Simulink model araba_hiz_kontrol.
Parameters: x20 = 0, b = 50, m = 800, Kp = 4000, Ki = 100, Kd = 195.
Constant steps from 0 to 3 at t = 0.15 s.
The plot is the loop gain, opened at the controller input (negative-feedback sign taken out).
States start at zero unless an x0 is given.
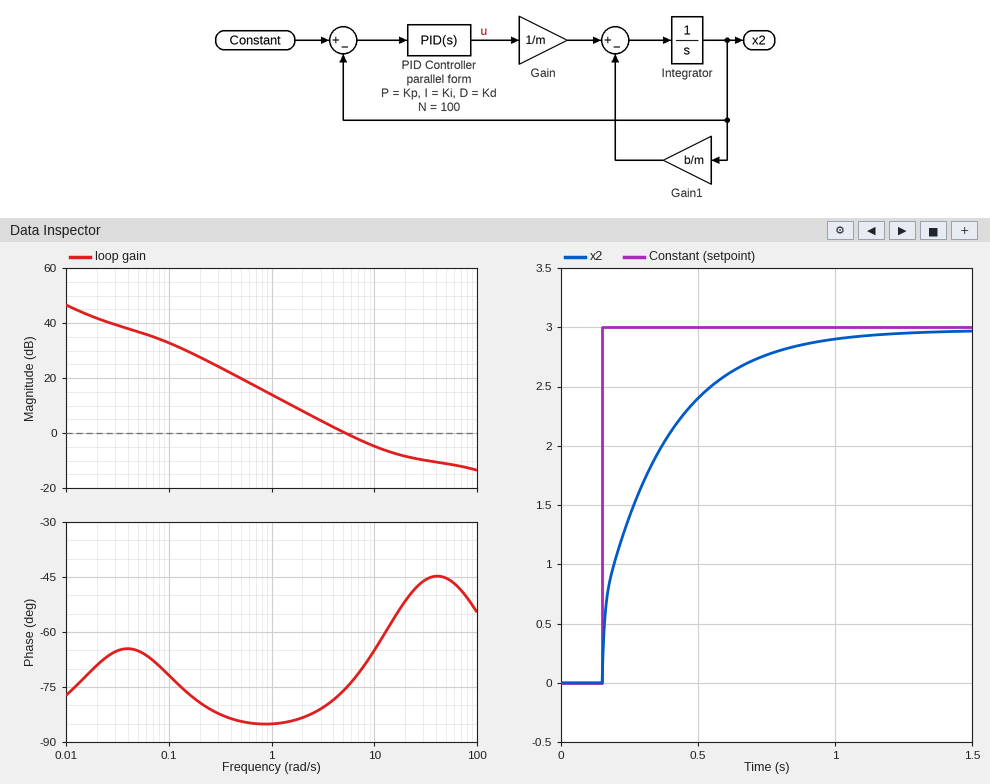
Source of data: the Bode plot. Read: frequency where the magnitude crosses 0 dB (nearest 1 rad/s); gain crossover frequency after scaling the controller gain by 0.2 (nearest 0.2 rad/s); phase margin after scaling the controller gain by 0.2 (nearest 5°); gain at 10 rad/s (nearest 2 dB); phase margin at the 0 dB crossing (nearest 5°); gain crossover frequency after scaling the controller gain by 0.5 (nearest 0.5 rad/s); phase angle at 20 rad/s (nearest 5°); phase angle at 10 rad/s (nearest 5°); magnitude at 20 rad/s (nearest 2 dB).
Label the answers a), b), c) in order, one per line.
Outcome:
a) 5 rad/s
b) 1.0 rad/s
c) 95°
d) -4 dB
e) 105°
f) 2.5 rad/s
g) -50°
h) -65°
i) -8 dB
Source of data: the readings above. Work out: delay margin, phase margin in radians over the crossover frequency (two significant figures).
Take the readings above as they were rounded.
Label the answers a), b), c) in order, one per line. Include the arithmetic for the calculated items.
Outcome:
a) 105 × π / 180 / 5 = 0.37 s
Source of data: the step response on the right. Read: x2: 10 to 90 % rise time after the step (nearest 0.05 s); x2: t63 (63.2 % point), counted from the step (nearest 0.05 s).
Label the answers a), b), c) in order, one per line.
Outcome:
a) 0.50 s
b) 0.20 s
